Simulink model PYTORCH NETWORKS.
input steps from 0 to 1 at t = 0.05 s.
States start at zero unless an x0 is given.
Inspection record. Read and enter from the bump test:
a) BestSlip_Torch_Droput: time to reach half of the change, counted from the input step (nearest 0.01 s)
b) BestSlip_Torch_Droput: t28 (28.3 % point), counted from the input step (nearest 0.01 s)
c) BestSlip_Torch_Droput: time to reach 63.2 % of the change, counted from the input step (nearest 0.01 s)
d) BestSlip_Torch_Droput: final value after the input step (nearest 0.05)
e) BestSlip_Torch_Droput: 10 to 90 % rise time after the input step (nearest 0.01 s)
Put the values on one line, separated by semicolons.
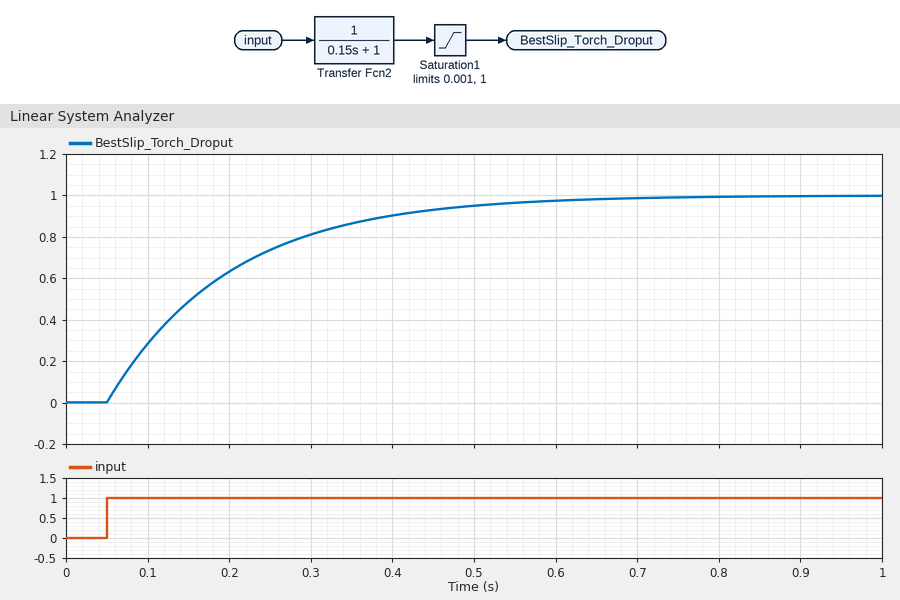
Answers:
0.10 s; 0.05 s; 0.15 s; 1.00; 0.33 s
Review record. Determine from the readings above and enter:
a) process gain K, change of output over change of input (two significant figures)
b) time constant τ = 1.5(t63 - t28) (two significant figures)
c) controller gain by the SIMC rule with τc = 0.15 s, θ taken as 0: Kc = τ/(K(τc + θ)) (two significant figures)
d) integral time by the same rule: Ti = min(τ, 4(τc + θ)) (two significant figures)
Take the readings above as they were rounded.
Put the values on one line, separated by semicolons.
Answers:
1.0; 0.15 s; 1.0; 0.15 s
